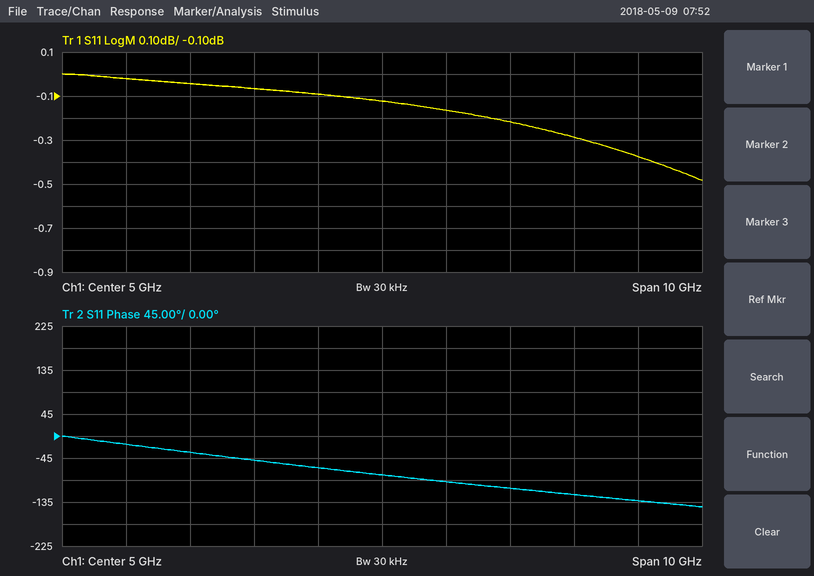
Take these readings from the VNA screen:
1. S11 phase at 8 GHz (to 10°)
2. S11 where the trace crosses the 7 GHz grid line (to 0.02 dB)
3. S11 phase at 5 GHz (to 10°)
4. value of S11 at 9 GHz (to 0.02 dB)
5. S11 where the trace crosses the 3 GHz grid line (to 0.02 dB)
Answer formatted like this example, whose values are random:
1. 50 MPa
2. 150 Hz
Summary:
1. -120°
2. -0.22 dB
3. -80°
4. -0.38 dB
5. -0.06 dB
